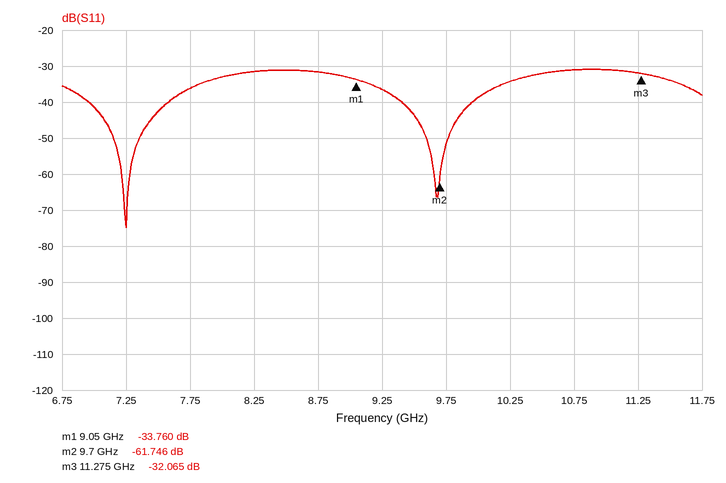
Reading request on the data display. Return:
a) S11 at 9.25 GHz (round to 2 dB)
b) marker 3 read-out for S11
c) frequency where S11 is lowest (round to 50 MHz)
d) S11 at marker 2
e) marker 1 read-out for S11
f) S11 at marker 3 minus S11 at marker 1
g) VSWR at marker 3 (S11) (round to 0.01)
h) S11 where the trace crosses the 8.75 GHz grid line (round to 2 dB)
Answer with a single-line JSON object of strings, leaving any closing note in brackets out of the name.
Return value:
{"S11 at 9.25 GHz": "-36 dB", "marker 3 read-out for S11": "-32.065 dB", "frequency where S11 is lowest": "7.25 GHz", "S11 at marker 2": "-61.746 dB", "marker 1 read-out for S11": "-33.760 dB", "S11 at marker 3 minus S11 at marker 1": "1.695 dB", "VSWR at marker 3 (S11)": "1.05", "S11 where the trace crosses the 8.75 GHz grid line": "-32 dB"}
